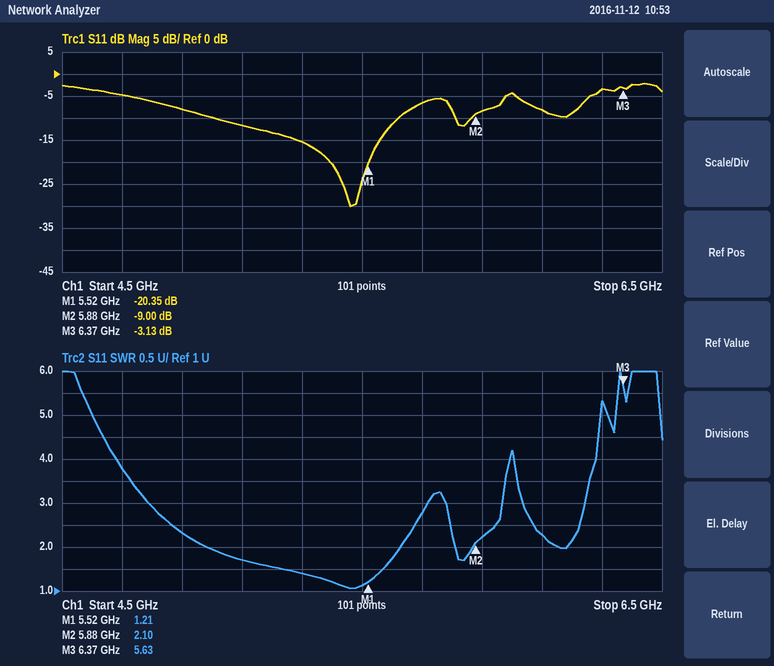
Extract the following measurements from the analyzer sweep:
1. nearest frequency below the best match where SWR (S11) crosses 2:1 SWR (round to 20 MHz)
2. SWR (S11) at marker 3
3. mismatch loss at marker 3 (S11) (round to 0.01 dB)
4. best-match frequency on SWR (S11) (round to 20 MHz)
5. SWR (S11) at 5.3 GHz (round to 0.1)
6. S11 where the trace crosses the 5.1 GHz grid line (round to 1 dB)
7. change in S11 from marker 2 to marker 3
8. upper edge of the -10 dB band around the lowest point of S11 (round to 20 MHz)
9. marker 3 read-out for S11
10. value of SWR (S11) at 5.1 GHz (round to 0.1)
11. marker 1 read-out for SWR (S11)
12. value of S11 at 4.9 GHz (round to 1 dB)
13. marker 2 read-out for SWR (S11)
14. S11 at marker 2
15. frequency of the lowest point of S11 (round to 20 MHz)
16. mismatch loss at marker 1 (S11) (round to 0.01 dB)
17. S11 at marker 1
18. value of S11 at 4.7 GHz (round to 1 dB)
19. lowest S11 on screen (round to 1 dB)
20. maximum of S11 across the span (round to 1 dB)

4.98 GHz
5.63
2.89 dB
5.46 GHz
1.4
-12 dB
5.87 dB
5.62 GHz
-3.13 dB
1.7
1.21
-8 dB
2.10
-9.00 dB
5.46 GHz
0.04 dB
-20.35 dB
-5 dB
-30 dB
-2 dB
